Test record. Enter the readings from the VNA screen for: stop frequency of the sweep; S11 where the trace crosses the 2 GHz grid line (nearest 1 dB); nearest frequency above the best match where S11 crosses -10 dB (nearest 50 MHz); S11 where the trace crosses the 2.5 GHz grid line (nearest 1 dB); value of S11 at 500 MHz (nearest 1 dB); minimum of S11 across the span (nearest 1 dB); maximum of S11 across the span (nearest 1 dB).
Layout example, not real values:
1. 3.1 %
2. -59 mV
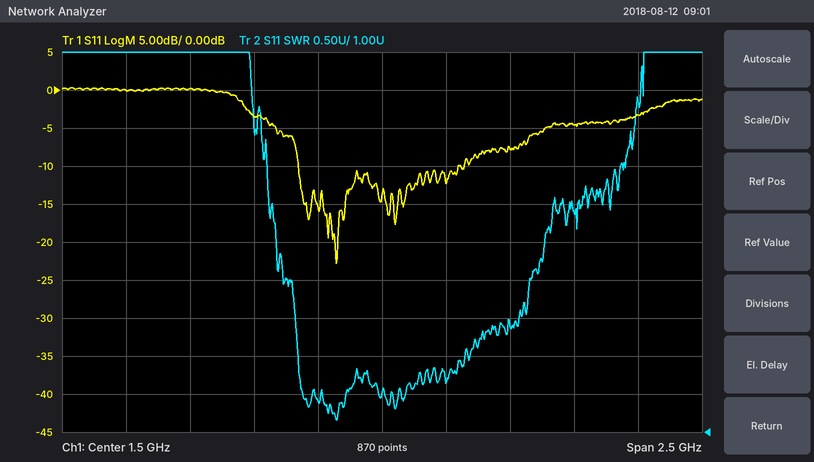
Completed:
1. 2.75 GHz
2. -8 dB
3. 1.80 GHz
4. -3 dB
5. 0 dB
6. -23 dB
7. 0 dB
